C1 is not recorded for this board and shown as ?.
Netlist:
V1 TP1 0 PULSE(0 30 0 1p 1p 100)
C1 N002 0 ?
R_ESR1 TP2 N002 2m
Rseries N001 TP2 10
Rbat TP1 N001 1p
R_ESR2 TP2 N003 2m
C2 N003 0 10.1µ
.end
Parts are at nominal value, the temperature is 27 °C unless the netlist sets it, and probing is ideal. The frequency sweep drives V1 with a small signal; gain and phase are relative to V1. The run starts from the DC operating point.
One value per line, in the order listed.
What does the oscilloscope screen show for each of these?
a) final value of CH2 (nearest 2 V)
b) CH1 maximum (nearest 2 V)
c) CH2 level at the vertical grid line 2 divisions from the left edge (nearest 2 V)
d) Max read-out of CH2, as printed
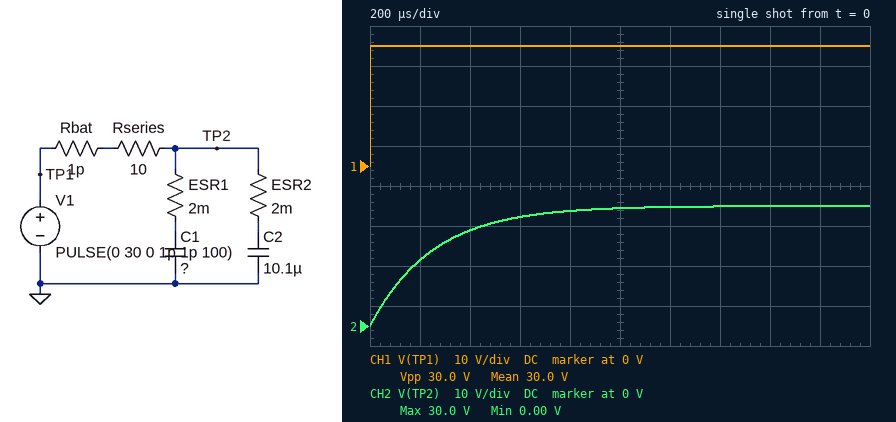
30 V
30 V
24 V
30.0 V
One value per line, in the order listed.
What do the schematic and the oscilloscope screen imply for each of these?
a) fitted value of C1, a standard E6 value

15 µF
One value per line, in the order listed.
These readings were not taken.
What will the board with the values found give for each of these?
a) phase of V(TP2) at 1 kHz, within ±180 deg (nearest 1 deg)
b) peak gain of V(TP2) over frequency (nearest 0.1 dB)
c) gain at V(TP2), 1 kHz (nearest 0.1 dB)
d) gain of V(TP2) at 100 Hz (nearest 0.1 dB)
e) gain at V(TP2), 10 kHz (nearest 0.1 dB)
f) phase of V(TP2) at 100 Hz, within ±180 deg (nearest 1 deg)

-58 deg
0 dB
-5.4 dB
-0.1 dB
-24.0 dB
-9 deg
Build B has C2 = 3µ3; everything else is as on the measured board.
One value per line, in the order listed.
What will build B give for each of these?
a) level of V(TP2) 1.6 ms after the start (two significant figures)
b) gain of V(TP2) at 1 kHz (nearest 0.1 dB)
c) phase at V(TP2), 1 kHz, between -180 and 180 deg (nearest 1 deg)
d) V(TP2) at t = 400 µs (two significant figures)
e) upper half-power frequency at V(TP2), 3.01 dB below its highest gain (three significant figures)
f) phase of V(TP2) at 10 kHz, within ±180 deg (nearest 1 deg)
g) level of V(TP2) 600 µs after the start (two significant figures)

30 V
-3.7 dB
-49 deg
27 V
870 Hz
-85 deg
29 V
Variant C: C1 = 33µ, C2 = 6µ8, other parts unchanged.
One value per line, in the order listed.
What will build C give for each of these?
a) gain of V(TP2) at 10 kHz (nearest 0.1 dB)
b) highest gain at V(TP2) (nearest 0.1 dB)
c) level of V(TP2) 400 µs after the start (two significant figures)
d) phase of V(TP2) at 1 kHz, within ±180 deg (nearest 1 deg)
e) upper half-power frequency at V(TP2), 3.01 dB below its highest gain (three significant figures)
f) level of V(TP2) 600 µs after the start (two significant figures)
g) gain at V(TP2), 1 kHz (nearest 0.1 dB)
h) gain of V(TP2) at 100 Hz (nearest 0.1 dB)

-28.0 dB
0 dB
19 V
-68 deg
400 Hz
23 V
-8.6 dB
-0.3 dB
